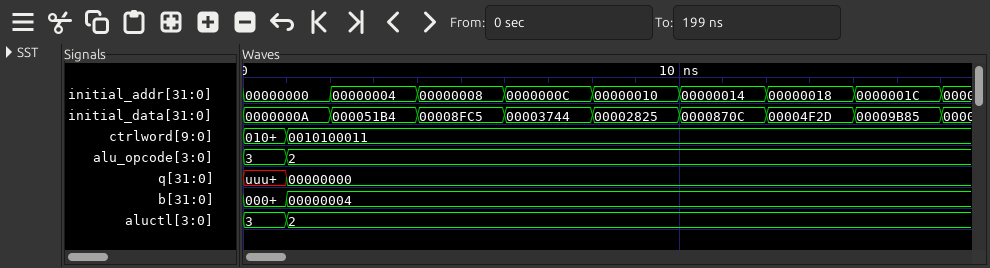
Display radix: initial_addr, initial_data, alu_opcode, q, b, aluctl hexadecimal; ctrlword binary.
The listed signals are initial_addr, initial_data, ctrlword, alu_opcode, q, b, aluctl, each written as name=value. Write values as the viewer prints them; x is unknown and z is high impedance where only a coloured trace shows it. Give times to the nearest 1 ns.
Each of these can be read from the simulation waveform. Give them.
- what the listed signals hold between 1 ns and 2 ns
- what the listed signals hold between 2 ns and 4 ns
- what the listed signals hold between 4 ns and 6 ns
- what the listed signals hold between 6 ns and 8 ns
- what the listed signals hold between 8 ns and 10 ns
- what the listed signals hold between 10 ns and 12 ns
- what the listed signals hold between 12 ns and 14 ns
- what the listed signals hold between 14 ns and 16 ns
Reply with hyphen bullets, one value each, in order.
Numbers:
- initial_addr=00000000, initial_data=0000000A, ctrlword=0010100011, alu_opcode=2, q=00000000, b=00000004, aluctl=2
- initial_addr=00000004, initial_data=000051B4, ctrlword=0010100011, alu_opcode=2, q=00000000, b=00000004, aluctl=2
- initial_addr=00000008, initial_data=00008FC5, ctrlword=0010100011, alu_opcode=2, q=00000000, b=00000004, aluctl=2
- initial_addr=0000000C, initial_data=00003744, ctrlword=0010100011, alu_opcode=2, q=00000000, b=00000004, aluctl=2
- initial_addr=00000010, initial_data=00002825, ctrlword=0010100011, alu_opcode=2, q=00000000, b=00000004, aluctl=2
- initial_addr=00000014, initial_data=0000870C, ctrlword=0010100011, alu_opcode=2, q=00000000, b=00000004, aluctl=2
- initial_addr=00000018, initial_data=00004F2D, ctrlword=0010100011, alu_opcode=2, q=00000000, b=00000004, aluctl=2
- initial_addr=0000001C, initial_data=00009B85, ctrlword=0010100011, alu_opcode=2, q=00000000, b=00000004, aluctl=2
